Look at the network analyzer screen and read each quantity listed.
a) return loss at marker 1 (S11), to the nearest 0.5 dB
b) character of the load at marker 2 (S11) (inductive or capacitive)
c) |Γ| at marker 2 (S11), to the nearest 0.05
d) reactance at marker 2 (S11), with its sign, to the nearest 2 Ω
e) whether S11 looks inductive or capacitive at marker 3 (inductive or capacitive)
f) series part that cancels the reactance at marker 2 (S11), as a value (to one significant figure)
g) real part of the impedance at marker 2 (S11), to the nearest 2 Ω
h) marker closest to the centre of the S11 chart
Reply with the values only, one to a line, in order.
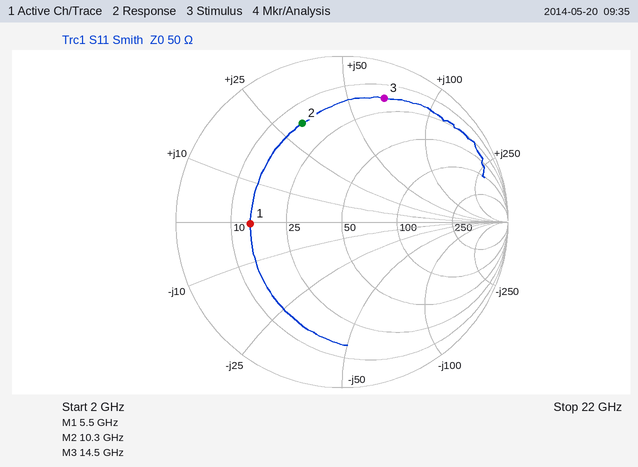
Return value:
5.0 dB
inductive
0.65
+32 Ω
inductive
500 fF
16 Ω
marker 1
